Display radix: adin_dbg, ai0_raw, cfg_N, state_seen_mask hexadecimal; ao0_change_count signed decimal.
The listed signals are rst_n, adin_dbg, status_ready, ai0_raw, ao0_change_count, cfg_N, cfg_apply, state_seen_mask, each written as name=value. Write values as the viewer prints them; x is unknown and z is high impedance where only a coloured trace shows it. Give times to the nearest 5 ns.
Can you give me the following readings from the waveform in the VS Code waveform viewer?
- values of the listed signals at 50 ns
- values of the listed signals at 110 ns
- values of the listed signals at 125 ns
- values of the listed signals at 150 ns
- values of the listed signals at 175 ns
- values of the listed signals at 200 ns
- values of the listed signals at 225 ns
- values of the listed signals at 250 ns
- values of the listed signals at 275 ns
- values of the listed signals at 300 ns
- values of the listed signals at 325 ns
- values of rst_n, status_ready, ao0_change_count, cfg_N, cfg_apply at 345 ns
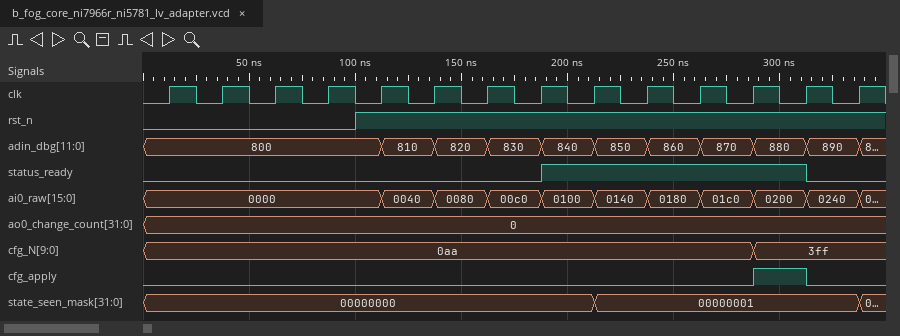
rst_n=0, adin_dbg=800, status_ready=0, ai0_raw=0000, ao0_change_count=0, cfg_N=0aa, cfg_apply=0, state_seen_mask=00000000
rst_n=1, adin_dbg=800, status_ready=0, ai0_raw=0000, ao0_change_count=0, cfg_N=0aa, cfg_apply=0, state_seen_mask=00000000
rst_n=1, adin_dbg=810, status_ready=0, ai0_raw=0040, ao0_change_count=0, cfg_N=0aa, cfg_apply=0, state_seen_mask=00000000
rst_n=1, adin_dbg=820, status_ready=0, ai0_raw=0080, ao0_change_count=0, cfg_N=0aa, cfg_apply=0, state_seen_mask=00000000
rst_n=1, adin_dbg=830, status_ready=0, ai0_raw=00c0, ao0_change_count=0, cfg_N=0aa, cfg_apply=0, state_seen_mask=00000000
rst_n=1, adin_dbg=840, status_ready=1, ai0_raw=0100, ao0_change_count=0, cfg_N=0aa, cfg_apply=0, state_seen_mask=00000000
rst_n=1, adin_dbg=850, status_ready=1, ai0_raw=0140, ao0_change_count=0, cfg_N=0aa, cfg_apply=0, state_seen_mask=00000001
rst_n=1, adin_dbg=860, status_ready=1, ai0_raw=0180, ao0_change_count=0, cfg_N=0aa, cfg_apply=0, state_seen_mask=00000001
rst_n=1, adin_dbg=870, status_ready=1, ai0_raw=01c0, ao0_change_count=0, cfg_N=0aa, cfg_apply=0, state_seen_mask=00000001
rst_n=1, adin_dbg=880, status_ready=1, ai0_raw=0200, ao0_change_count=0, cfg_N=3ff, cfg_apply=1, state_seen_mask=00000001
rst_n=1, adin_dbg=890, status_ready=0, ai0_raw=0240, ao0_change_count=0, cfg_N=3ff, cfg_apply=0, state_seen_mask=00000001
rst_n=1, status_ready=0, ao0_change_count=0, cfg_N=3ff, cfg_apply=0
